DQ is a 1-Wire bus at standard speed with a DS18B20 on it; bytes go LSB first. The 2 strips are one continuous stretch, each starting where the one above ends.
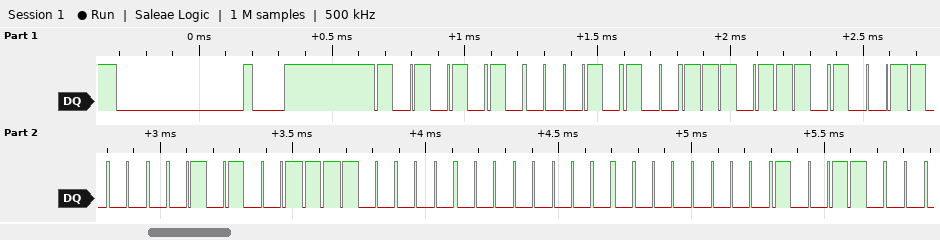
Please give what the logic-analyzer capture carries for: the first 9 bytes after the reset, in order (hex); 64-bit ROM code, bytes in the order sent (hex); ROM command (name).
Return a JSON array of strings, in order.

["55 28 77 19 94 07 00 00 19", "28 77 19 94 07 00 00 19", "Match ROM"]
